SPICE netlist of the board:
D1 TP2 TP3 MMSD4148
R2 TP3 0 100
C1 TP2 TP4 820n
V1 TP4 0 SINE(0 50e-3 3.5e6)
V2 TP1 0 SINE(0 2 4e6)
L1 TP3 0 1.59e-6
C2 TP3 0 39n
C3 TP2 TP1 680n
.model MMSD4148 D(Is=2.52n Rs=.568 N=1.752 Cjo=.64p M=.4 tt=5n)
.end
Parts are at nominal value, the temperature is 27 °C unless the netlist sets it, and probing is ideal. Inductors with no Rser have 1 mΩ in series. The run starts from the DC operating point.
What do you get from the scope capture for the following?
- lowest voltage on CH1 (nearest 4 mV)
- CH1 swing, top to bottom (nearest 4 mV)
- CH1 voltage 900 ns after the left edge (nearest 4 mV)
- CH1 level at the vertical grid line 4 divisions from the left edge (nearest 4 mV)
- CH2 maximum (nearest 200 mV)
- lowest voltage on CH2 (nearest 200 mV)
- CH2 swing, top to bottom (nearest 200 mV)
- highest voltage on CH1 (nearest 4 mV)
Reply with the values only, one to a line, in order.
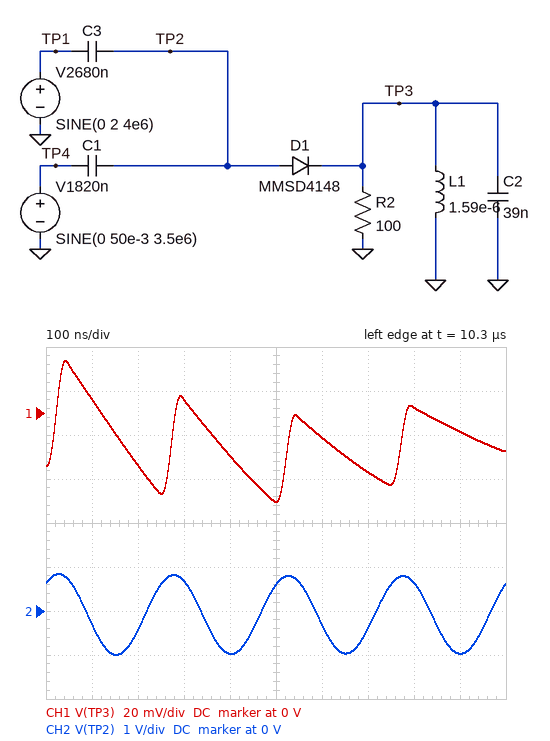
-40 mV
64 mV
-8 mV
-20 mV
800 mV
-1.0 V
1.8 V
24 mV
